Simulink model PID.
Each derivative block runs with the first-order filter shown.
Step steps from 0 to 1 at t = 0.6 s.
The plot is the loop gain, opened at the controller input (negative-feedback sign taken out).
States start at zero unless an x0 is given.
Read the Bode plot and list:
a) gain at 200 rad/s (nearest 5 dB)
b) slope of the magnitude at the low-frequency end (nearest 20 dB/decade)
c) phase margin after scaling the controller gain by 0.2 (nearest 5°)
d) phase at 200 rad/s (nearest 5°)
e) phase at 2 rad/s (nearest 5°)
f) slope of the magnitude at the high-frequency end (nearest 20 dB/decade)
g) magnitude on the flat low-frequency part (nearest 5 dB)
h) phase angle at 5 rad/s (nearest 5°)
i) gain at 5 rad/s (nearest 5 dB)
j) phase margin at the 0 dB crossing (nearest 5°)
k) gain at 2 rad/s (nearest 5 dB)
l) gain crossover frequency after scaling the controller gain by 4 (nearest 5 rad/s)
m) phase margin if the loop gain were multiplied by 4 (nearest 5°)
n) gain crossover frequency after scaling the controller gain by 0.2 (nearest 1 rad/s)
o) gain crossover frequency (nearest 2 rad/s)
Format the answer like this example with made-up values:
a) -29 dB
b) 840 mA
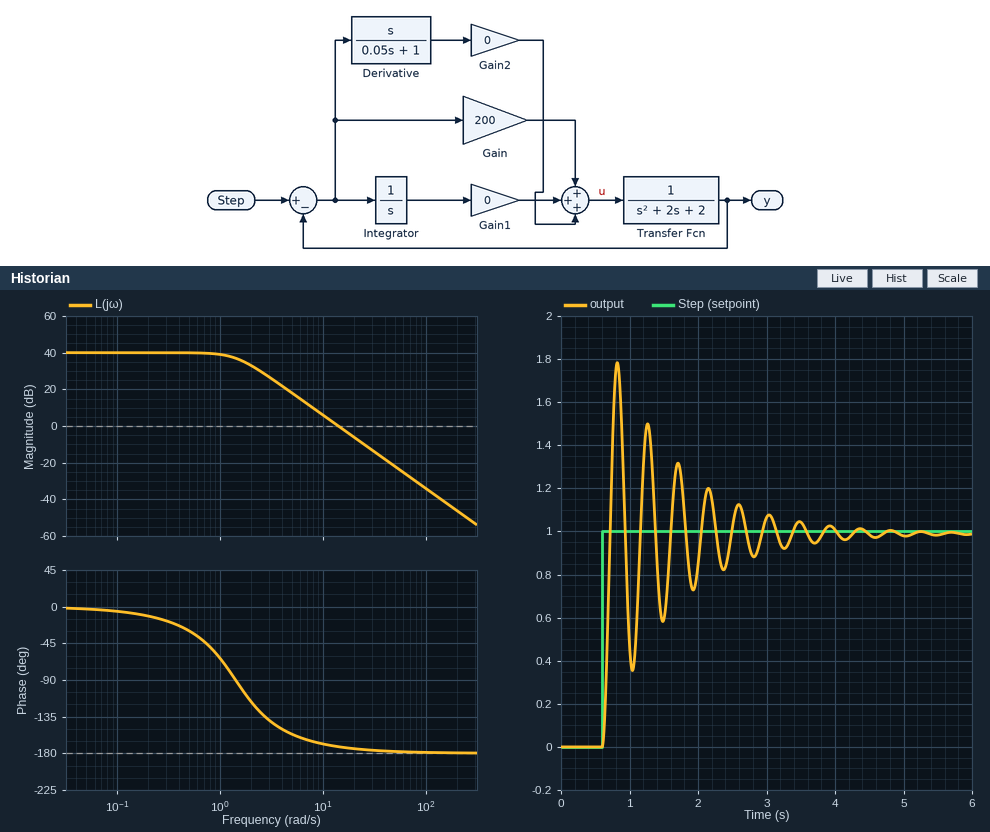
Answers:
a) -45 dB
b) 0 dB/decade
c) 20°
d) -180°
e) -115°
f) -40 dB/decade
g) 40 dB
h) -155°
i) 20 dB
j) 10°
k) 35 dB
l) 30 rad/s
m) 5°
n) 6 rad/s
o) 14 rad/s
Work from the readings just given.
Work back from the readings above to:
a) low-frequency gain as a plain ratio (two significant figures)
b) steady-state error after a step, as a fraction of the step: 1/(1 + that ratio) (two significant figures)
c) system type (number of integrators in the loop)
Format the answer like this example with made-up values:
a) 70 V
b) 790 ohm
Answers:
a) 100
b) 0.0099
c) 0
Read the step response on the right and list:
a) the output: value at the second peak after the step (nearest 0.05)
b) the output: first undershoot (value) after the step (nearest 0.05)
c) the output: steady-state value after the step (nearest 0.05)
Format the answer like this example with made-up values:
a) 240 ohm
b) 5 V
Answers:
a) 1.50
b) 0.35
c) 1.00
